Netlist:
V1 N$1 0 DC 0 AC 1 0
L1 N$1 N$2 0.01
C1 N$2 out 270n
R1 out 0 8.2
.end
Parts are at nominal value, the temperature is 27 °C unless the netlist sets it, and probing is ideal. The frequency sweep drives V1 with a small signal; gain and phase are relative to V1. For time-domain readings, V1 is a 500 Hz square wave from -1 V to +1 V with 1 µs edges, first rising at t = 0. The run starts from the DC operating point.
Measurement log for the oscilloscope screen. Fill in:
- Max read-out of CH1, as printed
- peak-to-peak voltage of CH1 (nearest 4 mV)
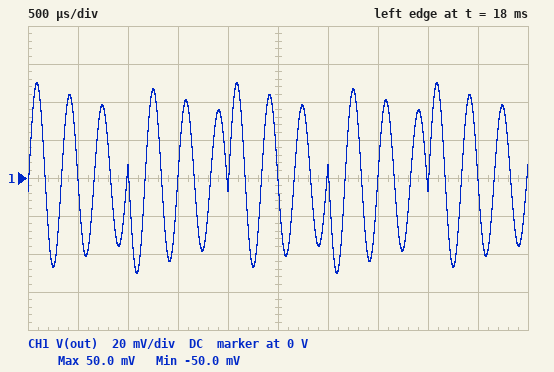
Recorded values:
50.0 mV
100 mV
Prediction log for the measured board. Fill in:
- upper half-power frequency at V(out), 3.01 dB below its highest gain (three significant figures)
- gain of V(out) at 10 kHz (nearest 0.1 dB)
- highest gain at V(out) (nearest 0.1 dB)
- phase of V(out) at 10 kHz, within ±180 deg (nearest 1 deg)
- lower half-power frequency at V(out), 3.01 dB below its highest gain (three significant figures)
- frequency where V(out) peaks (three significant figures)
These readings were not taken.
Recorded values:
3.13 kHz
-36.8 dB
0 dB
-89 deg
3.00 kHz
3.06 kHz
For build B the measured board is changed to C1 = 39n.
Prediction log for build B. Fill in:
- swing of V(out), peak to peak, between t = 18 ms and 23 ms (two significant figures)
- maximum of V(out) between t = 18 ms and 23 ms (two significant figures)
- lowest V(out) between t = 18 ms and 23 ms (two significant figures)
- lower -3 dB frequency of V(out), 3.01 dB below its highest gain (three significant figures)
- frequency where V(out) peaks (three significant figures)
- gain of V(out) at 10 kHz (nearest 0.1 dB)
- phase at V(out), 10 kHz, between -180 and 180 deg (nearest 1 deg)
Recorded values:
39 mV
19 mV
-19 mV
7.99 kHz
8.06 kHz
-28.6 dB
-88 deg
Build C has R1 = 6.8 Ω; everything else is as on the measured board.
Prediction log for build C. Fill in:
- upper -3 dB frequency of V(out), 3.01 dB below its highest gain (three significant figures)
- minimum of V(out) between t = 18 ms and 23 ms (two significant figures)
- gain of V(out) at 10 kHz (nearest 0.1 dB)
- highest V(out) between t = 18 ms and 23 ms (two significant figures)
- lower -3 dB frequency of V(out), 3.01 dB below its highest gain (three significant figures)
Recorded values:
3.12 kHz
-41 mV
-38.5 dB
41 mV
3.01 kHz
